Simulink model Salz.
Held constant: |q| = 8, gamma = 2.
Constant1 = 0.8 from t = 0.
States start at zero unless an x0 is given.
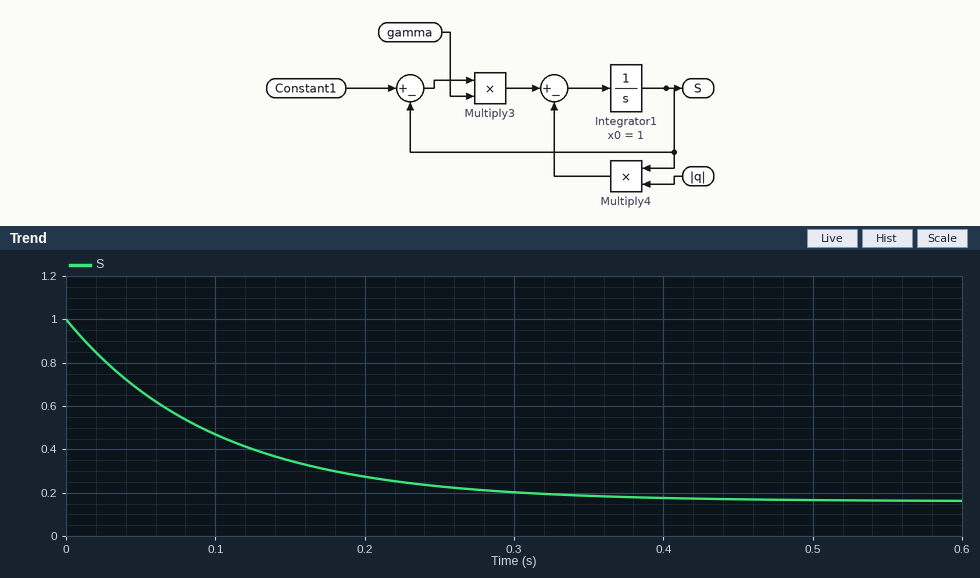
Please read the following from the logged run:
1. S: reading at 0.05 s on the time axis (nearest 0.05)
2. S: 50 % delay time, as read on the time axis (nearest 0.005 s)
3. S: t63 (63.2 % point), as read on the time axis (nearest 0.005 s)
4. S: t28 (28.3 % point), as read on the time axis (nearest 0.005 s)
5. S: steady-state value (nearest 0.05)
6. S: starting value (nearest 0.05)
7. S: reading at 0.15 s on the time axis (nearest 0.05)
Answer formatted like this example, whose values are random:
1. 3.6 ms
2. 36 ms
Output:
1. 0.65
2. 0.070 s
3. 0.100 s
4. 0.035 s
5. 0.15
6. 1.00
7. 0.35
